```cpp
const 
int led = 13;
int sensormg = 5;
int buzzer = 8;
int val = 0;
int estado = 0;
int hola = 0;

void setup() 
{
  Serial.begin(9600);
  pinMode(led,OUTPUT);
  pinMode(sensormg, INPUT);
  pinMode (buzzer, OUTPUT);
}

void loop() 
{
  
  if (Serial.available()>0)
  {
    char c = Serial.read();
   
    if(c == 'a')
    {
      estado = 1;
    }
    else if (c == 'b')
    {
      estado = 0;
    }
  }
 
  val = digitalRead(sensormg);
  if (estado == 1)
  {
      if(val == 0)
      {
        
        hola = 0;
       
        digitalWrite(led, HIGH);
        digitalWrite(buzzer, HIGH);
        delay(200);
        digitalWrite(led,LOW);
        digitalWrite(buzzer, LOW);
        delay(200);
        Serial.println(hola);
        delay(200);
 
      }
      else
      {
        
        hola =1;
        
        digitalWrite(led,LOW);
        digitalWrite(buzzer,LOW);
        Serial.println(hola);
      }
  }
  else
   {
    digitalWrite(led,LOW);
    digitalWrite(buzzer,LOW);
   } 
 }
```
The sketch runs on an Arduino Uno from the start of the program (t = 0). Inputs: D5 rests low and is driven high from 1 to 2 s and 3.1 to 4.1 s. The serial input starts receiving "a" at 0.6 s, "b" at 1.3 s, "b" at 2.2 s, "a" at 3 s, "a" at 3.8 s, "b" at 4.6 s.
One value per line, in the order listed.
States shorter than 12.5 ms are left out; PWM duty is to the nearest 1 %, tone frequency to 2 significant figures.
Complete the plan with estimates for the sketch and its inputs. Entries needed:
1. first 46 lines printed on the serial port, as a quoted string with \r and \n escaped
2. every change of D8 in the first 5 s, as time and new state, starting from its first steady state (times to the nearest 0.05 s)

"0\r\n1\r\n1\r\n1\r\n1\r\n1\r\n1\r\n1\r\n1\r\n1\r\n1\r\n1\r\n1\r\n1\r\n1\r\n1\r\n1\r\n1\r\n1\r\n1\r\n1\r\n1\r\n1\r\n1\r\n1\r\n1\r\n1\r\n1\r\n1\r\n1\r\n1\r\n1\r\n1\r\n1\r\n1\r\n1\r\n1\r\n1\r\n1\r\n1\r\n1\r\n1\r\n1\r\n1\r\n1\r\n1\r\n"
0 s low; 0.6 s high; 0.8 s low; 3 s high; 3.2 s low; 4.1 s high; 4.3 s low
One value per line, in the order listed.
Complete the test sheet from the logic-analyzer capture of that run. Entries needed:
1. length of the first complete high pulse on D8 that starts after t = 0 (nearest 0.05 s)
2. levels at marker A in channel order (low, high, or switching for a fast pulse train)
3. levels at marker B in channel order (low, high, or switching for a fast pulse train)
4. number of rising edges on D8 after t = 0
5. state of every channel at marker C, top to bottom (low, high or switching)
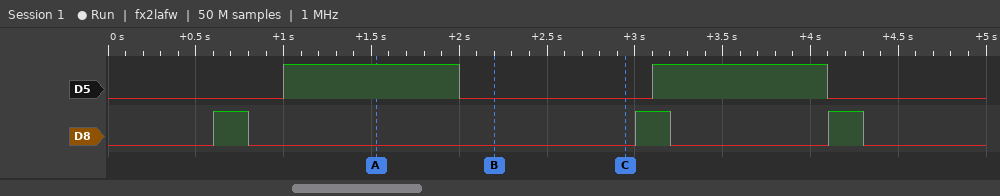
0.20 s
D5 high, D8 low
D5 low, D8 low
3
D5 low, D8 low
